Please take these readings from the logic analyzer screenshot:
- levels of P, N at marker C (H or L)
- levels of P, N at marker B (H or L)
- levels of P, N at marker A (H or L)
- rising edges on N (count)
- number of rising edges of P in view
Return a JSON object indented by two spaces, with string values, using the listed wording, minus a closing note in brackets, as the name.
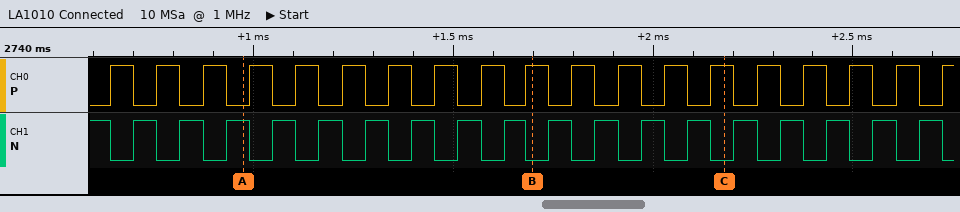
{
  "levels of P, N at marker C": "P=H, N=L",
  "levels of P, N at marker B": "P=H, N=L",
  "levels of P, N at marker A": "P=L, N=H",
  "rising edges on N": "18",
  "number of rising edges of P in view": "19"
}
